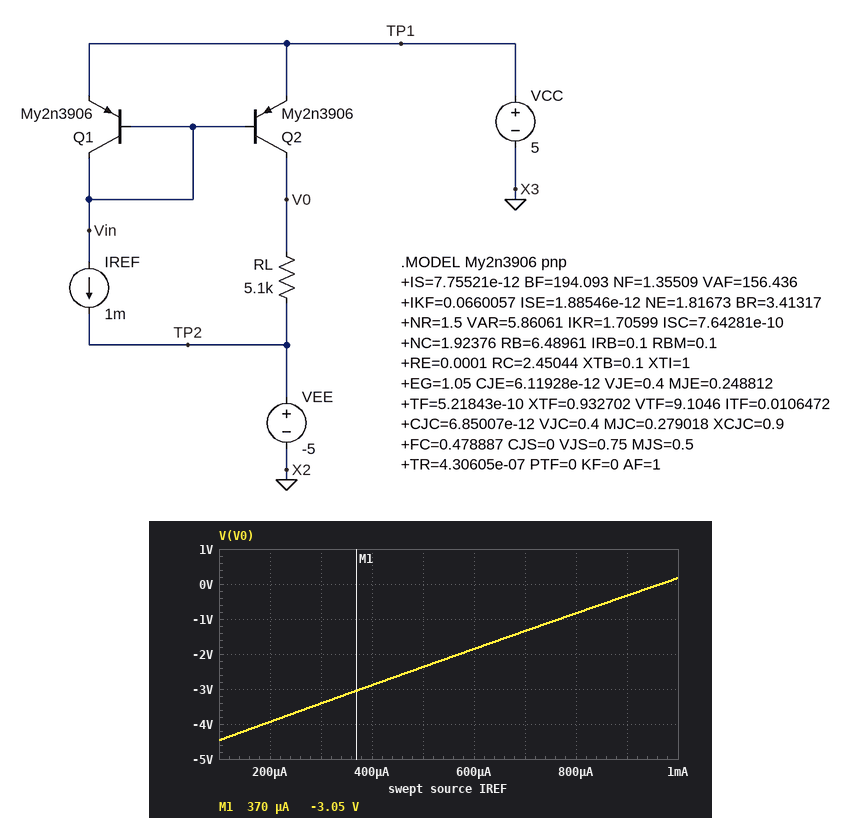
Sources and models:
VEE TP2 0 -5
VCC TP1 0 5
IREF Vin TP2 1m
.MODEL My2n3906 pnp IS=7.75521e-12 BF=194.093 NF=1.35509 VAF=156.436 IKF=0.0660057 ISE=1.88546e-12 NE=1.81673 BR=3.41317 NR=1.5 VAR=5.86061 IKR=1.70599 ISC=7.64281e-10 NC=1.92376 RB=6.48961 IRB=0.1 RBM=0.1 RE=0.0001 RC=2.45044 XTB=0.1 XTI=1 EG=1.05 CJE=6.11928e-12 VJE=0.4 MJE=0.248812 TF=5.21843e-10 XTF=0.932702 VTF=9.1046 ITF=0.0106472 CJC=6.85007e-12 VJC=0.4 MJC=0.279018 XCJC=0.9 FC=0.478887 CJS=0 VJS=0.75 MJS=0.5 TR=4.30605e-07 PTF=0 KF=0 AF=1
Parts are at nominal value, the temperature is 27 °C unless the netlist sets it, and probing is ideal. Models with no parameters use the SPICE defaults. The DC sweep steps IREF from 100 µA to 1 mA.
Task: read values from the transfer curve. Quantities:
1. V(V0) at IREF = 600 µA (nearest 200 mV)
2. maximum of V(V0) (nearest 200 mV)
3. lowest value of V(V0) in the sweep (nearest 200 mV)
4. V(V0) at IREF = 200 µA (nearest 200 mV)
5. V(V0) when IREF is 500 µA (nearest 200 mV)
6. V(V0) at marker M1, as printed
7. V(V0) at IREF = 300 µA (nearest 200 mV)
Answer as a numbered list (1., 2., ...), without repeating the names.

1. -1.8 V
2. 200 mV
3. -4.4 V
4. -4.0 V
5. -2.4 V
6. -3.05 V
7. -3.4 V
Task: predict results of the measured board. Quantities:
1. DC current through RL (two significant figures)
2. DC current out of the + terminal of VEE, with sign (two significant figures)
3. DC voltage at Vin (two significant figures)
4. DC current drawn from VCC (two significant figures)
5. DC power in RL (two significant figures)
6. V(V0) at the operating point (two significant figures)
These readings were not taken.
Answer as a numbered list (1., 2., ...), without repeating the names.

1. 1.0 mA
2. -2.0 mA
3. 4.3 V
4. 2.0 mA
5. 5.2 mW
6. 170 mV
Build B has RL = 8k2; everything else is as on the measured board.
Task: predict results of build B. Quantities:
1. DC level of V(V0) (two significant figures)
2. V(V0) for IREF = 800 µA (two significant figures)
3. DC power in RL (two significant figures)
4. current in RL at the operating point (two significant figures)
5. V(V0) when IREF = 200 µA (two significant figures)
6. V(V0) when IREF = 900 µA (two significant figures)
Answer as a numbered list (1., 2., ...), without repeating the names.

1. 3.1 V
2. 1.6 V
3. 8.1 mW
4. 990 µA
5. -3.3 V
6. 2.4 V
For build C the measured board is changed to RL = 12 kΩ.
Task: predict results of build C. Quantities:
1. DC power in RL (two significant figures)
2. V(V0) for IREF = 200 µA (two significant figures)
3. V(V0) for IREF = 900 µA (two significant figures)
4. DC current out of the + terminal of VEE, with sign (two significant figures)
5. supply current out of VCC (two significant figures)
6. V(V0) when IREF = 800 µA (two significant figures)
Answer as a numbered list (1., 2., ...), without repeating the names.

1. 8.2 mW
2. -2.5 V
3. 4.9 V
4. -1.8 mA
5. 1.8 mA
6. 4.4 V
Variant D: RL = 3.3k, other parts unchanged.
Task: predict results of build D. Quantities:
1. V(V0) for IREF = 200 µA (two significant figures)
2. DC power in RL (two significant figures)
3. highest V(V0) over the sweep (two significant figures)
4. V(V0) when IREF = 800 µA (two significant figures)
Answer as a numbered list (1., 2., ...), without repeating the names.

1. -4.3 V
2. 3.5 mW
3. -1.6 V
4. -2.3 V
